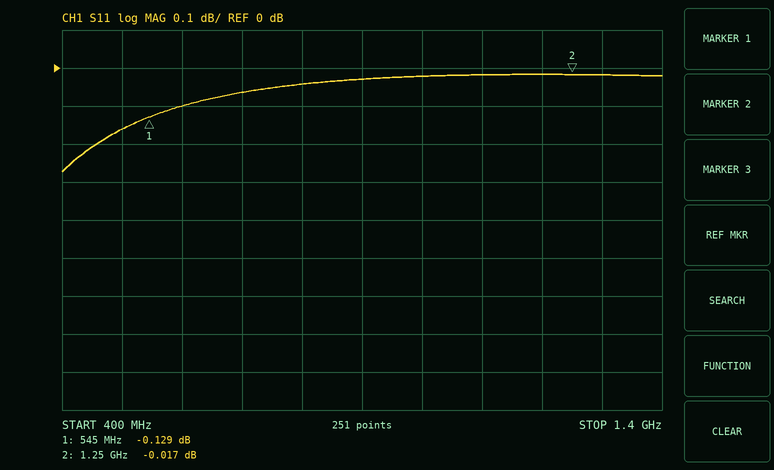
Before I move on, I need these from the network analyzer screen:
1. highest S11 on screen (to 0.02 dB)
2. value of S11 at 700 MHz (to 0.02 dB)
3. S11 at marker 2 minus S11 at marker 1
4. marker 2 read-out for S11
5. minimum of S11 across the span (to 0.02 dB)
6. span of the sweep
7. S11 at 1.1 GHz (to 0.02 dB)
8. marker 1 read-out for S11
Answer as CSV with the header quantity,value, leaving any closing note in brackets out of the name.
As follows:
quantity,value
highest S11 on screen,-0.02 dB
value of S11 at 700 MHz,-0.06 dB
S11 at marker 2 minus S11 at marker 1,0.112 dB
marker 2 read-out for S11,-0.017 dB
minimum of S11 across the span,-0.28 dB
span of the sweep,1 GHz
S11 at 1.1 GHz,-0.02 dB
marker 1 read-out for S11,-0.129 dB
